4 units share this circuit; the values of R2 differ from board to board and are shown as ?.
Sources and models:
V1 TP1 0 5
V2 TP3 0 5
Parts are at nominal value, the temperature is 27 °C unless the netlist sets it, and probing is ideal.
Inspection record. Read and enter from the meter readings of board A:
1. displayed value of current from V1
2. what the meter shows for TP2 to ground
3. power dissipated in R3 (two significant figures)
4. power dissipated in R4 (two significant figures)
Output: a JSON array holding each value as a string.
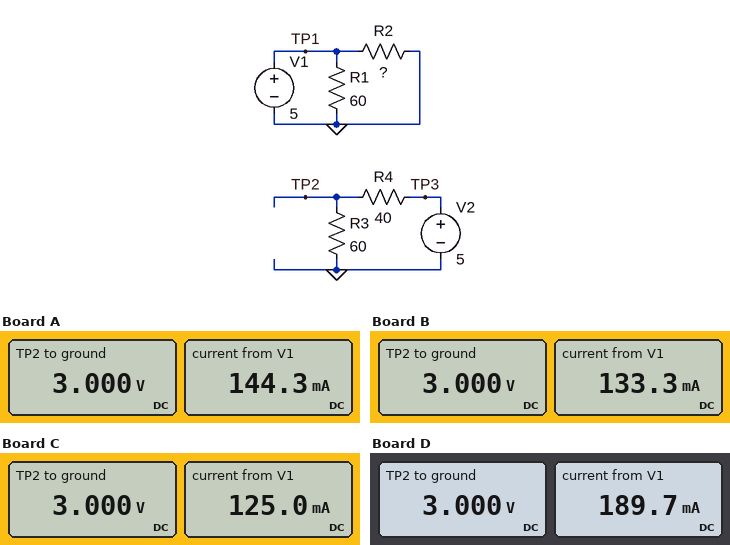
["144.3 mA", "3.000 V", "150 mW", "100 mW"]
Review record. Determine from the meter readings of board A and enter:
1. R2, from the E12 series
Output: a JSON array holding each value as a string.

["82 Ω"]
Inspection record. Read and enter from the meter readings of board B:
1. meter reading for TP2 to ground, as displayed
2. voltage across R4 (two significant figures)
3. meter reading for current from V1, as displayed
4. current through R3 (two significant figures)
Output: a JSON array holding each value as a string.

["3.000 V", "2.0 V", "133.3 mA", "50 mA"]
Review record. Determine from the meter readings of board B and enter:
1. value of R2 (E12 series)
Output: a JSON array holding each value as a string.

["100 Ω"]
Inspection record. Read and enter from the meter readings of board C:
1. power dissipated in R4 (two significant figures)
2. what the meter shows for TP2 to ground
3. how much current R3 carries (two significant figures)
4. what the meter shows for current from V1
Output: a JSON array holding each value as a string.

["100 mW", "3.000 V", "50 mA", "125.0 mA"]
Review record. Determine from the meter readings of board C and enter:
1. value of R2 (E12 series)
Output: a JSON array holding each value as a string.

["120 Ω"]
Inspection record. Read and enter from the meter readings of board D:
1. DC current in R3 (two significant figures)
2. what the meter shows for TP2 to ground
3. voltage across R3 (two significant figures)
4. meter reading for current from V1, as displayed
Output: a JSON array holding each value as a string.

["50 mA", "3.000 V", "3.0 V", "189.7 mA"]
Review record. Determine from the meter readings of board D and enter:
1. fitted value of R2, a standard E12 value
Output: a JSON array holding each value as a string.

["47 Ω"]
